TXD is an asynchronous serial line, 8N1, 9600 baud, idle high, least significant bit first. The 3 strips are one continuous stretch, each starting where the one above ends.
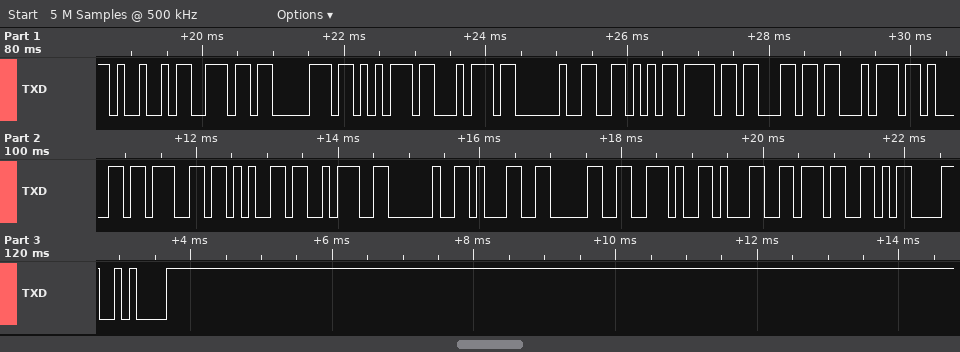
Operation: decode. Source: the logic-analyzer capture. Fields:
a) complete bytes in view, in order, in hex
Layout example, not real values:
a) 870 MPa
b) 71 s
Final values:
a) 49 6E 70 75 74 20 56 6F 6C 74 61 67 65 3A 20 31 30 2E 31 37 0D 0A
